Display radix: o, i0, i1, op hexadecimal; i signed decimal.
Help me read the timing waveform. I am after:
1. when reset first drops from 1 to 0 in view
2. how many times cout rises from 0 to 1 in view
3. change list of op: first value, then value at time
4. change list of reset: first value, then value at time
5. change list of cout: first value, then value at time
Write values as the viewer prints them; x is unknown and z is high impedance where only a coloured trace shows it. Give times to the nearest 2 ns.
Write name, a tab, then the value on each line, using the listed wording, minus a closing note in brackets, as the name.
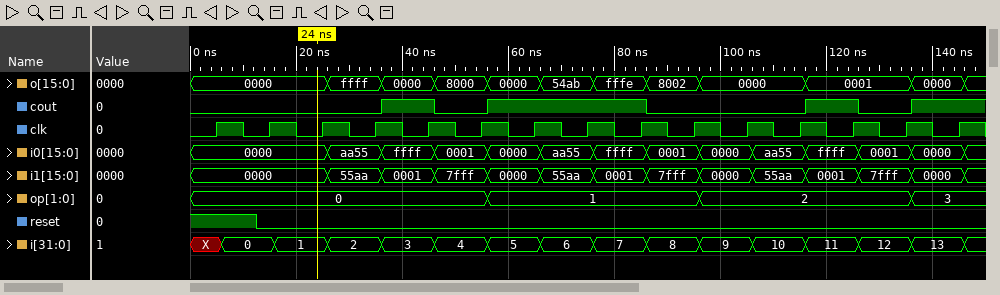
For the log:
when reset first drops from 1 to 0 in view	12 ns
how many times cout rises from 0 to 1 in view	4
change list of op: first value, then value at time	0, 1 at 56 ns, 2 at 96 ns, 3 at 136 ns
change list of reset: first value, then value at time	1, 0 at 12 ns
change list of cout: first value, then value at time	0, 1 at 36 ns, 0 at 46 ns, 1 at 56 ns, 0 at 86 ns, 1 at 116 ns, 0 at 126 ns, 1 at 136 ns
